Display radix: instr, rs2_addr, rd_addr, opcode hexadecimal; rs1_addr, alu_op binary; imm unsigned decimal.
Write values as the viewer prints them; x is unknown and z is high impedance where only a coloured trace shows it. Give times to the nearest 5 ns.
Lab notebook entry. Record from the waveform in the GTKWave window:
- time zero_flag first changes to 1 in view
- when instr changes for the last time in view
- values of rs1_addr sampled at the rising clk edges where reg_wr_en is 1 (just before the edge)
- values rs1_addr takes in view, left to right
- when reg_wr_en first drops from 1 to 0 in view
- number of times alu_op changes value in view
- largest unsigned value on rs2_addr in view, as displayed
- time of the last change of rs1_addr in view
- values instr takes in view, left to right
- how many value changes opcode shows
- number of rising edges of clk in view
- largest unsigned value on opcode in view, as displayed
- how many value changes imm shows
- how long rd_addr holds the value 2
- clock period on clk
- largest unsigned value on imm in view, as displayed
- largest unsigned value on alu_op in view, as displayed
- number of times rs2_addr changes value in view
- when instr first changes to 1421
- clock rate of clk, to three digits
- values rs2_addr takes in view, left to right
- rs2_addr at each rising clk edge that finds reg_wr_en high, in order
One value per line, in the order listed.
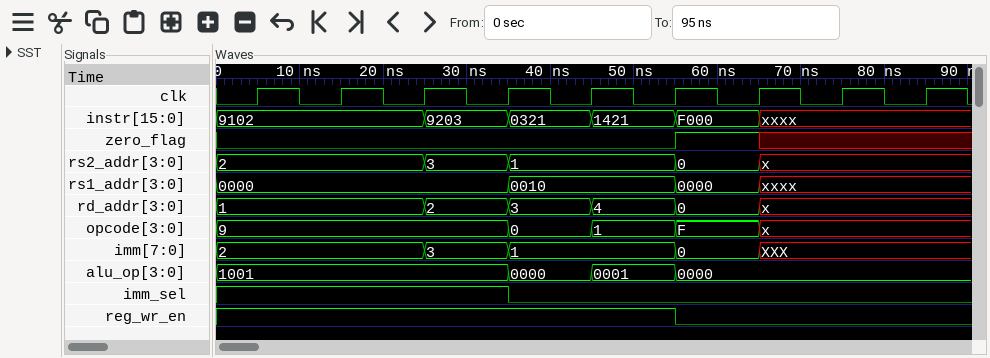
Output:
55 ns
65 ns
0000, 0000, 0000, 0000, 0010, 0010
0000, 0010, 0000, xxxx
55 ns
3
3
65 ns
9102, 9203, 0321, 1421, F000, xxxx
4
9
F
4
10 ns
10 ns
3
1001
4
45 ns
100 MHz
2, 3, 1, 0, x
2, 2, 2, 3, 1, 1
